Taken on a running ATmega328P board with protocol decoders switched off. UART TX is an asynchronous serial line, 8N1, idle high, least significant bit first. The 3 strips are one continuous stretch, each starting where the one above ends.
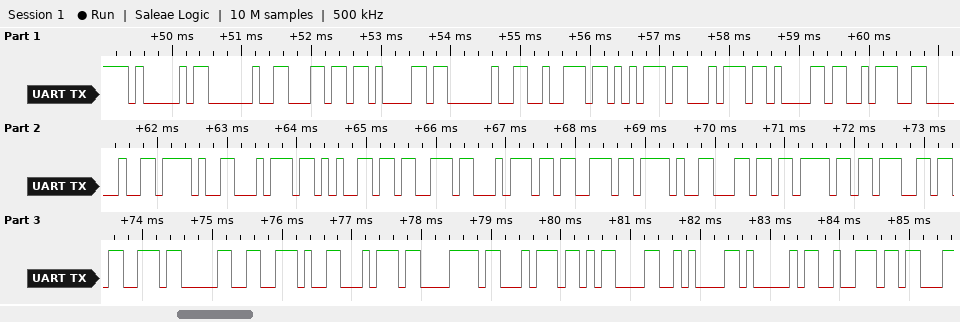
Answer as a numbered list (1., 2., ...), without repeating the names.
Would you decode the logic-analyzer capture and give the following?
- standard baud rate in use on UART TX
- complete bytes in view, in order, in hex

1. 9600 baud
2. 41 20 6C 61 20 72 75 74 61 3A 20 2F 74 65 73 74 73 2F 6C 6F 67 73 30 2E 74 78 74 0D 0A 41 72
